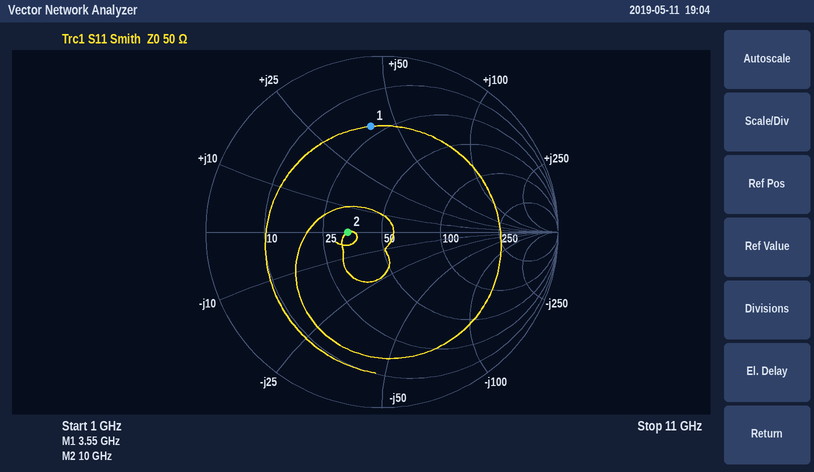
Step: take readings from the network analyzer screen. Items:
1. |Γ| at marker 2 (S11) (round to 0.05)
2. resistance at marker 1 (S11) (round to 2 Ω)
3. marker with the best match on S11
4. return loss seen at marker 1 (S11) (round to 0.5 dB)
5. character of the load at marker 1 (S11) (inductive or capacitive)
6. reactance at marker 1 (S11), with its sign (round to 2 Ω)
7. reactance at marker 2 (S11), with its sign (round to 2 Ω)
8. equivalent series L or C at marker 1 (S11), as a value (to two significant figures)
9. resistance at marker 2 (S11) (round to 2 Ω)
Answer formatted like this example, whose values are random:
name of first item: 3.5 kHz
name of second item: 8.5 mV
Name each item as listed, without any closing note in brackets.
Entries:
|Γ| at marker 2 (S11): 0.20
resistance at marker 1 (S11): 22 Ω
marker with the best match on S11: marker 2
return loss seen at marker 1 (S11): 4.5 dB
character of the load at marker 1 (S11): inductive
reactance at marker 1 (S11), with its sign: +40 Ω
reactance at marker 2 (S11), with its sign: 0 Ω
equivalent series L or C at marker 1 (S11), as a value: 1.8 nH
resistance at marker 2 (S11): 34 Ω
